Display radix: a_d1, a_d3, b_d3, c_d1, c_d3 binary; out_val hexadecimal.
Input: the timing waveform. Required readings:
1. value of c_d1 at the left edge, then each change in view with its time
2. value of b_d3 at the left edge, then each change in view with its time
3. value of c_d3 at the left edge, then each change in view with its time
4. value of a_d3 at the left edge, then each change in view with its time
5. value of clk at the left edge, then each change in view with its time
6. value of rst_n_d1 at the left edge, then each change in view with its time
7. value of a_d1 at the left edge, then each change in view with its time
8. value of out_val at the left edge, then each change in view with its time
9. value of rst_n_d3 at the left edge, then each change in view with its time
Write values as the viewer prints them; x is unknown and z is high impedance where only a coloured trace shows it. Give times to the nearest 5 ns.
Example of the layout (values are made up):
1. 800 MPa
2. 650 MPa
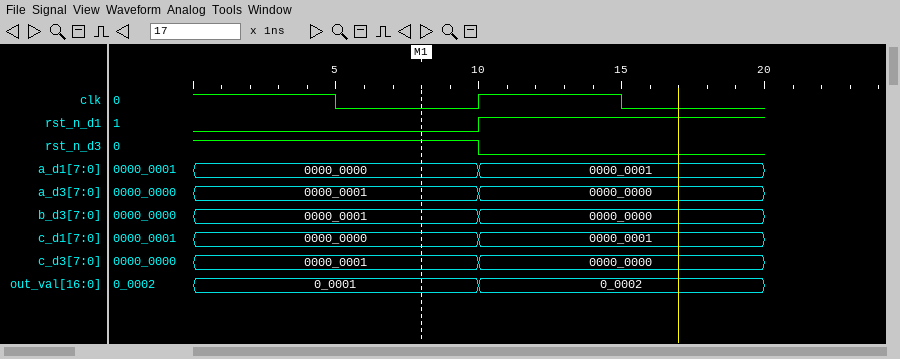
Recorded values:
1. 0000_0000, 0000_0001 at 10 ns
2. 0000_0001, 0000_0000 at 10 ns
3. 0000_0001, 0000_0000 at 10 ns
4. 0000_0001, 0000_0000 at 10 ns
5. 1, 0 at 5 ns, 1 at 10 ns, 0 at 15 ns
6. 0, 1 at 10 ns
7. 0000_0000, 0000_0001 at 10 ns
8. 0_0001, 0_0002 at 10 ns
9. 1, 0 at 10 ns
